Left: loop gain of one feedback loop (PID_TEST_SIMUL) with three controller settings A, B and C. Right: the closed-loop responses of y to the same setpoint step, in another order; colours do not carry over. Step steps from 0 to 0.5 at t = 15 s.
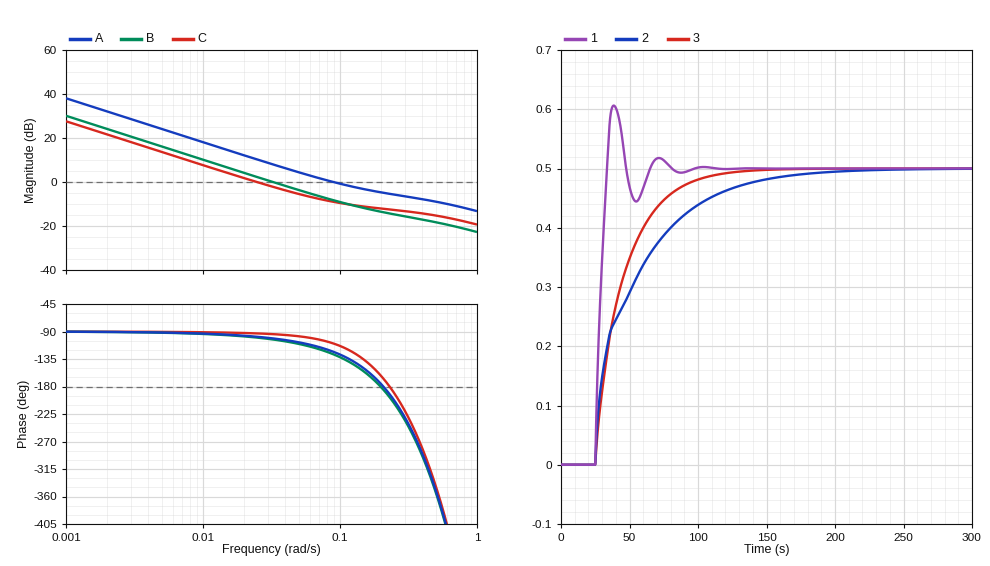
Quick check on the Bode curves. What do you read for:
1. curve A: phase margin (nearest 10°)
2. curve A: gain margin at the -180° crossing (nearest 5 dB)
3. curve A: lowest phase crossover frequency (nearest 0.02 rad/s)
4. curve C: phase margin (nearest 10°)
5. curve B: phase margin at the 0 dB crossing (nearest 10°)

60°
5 dB
0.20 rad/s
90°
80°
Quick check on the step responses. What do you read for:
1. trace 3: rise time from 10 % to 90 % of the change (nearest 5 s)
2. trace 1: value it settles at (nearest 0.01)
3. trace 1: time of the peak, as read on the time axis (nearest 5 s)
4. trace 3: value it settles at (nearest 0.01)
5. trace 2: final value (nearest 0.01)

50 s
0.50
40 s
0.50
0.50
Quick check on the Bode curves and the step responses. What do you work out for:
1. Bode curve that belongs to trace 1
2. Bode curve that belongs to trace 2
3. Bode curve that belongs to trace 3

A
C
B
